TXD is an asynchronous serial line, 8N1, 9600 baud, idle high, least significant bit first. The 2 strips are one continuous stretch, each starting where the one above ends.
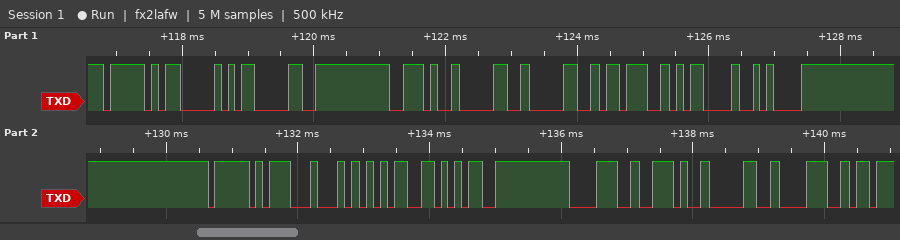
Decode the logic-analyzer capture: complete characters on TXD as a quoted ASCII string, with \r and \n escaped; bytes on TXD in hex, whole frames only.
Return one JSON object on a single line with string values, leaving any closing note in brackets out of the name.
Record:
{"complete characters on TXD as a quoted ASCII string, with \\r and \\n escaped": "\"_P0.00;\\r\\n_D558.08\"", "bytes on TXD in hex, whole frames only": "5F 50 30 2E 30 30 3B 0D 0A 5F 44 35 35 38 2E 30 38"}
